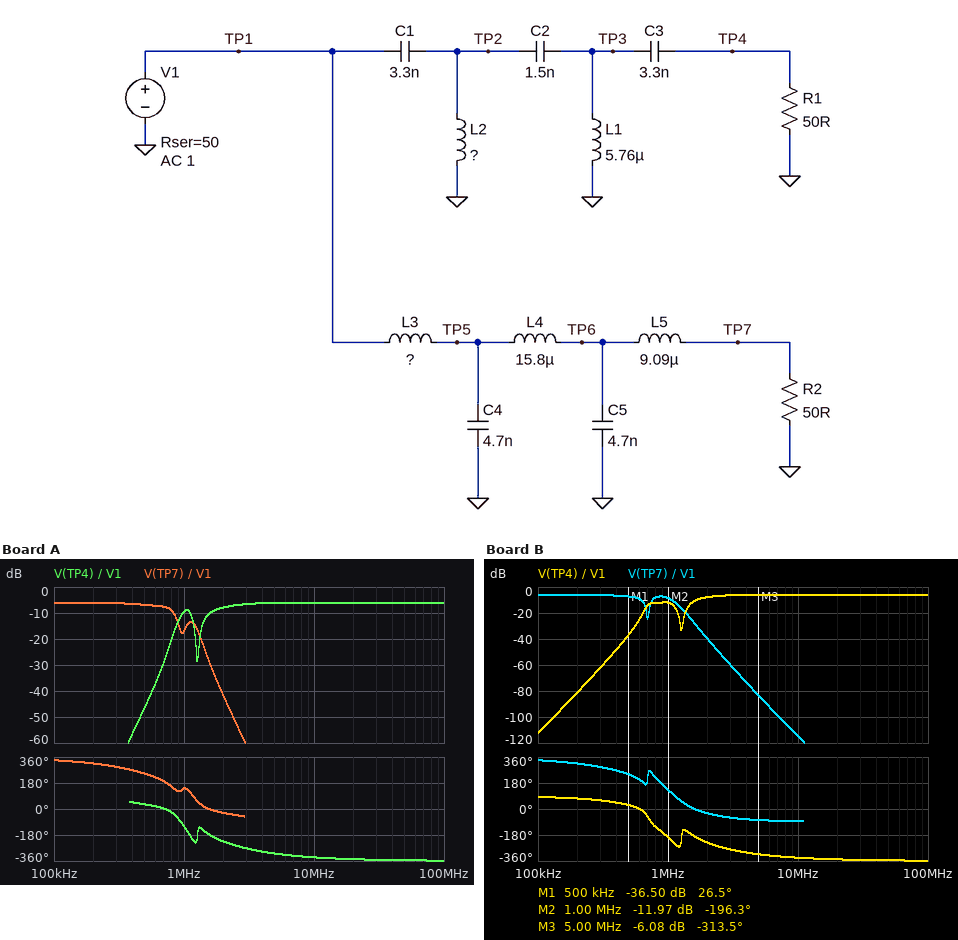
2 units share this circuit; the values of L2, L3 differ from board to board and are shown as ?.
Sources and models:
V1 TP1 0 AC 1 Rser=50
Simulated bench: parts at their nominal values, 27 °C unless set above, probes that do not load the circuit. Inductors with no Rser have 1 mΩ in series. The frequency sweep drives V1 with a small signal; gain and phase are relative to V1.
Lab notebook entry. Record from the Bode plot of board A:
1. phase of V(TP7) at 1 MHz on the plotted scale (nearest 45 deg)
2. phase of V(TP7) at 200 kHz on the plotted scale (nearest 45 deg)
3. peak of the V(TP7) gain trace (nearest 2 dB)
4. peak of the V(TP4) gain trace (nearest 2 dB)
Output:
135 deg
315 deg
-6 dB
-6 dB
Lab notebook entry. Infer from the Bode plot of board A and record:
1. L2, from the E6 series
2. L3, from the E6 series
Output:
4.7 µH
4.7 µH
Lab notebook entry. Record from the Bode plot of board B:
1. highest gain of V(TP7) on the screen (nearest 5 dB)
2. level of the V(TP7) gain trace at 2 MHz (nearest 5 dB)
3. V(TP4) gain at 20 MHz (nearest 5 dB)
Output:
-5 dB
-40 dB
-5 dB
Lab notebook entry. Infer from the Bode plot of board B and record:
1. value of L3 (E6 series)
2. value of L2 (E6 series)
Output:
4.7 µH
10 µH
